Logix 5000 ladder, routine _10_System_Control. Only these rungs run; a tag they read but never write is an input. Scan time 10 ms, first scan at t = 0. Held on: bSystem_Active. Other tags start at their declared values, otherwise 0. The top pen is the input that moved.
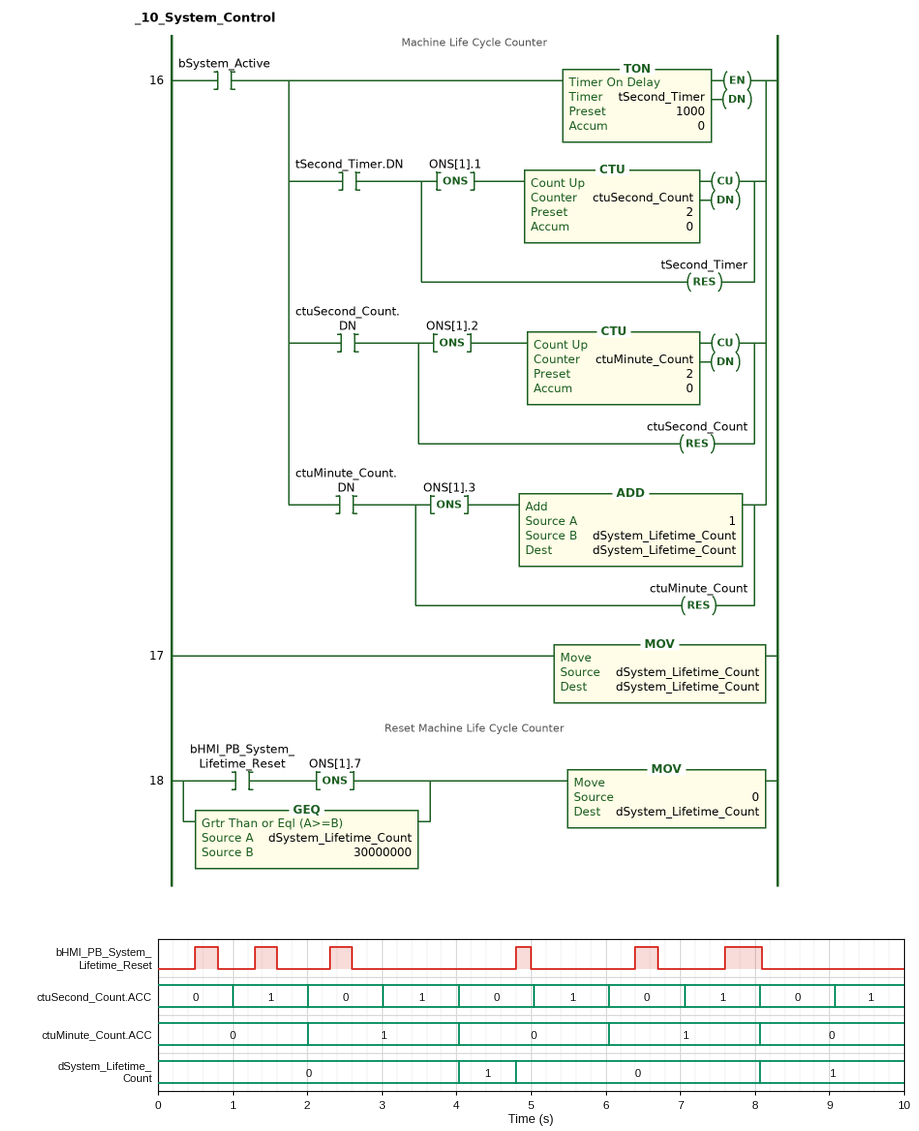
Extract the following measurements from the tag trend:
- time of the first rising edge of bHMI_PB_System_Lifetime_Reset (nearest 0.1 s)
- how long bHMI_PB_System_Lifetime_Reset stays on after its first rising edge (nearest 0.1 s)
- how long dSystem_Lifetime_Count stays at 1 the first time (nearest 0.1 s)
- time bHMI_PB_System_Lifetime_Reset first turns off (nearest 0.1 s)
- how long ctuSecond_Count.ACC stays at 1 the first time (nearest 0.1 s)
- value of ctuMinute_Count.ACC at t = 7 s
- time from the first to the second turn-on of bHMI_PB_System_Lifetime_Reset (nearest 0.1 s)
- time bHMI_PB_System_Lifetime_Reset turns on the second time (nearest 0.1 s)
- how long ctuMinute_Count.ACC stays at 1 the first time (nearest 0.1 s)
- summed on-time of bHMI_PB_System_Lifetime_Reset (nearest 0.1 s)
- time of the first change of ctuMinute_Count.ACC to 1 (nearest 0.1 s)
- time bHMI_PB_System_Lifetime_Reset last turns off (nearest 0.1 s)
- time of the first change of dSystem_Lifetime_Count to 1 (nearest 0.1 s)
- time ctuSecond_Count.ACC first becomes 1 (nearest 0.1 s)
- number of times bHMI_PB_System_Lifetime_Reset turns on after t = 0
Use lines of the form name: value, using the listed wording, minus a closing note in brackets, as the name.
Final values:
time of the first rising edge of bHMI_PB_System_Lifetime_Reset: 0.5 s
how long bHMI_PB_System_Lifetime_Reset stays on after its first rising edge: 0.3 s
how long dSystem_Lifetime_Count stays at 1 the first time: 0.8 s
time bHMI_PB_System_Lifetime_Reset first turns off: 0.8 s
how long ctuSecond_Count.ACC stays at 1 the first time: 1.0 s
value of ctuMinute_Count.ACC at t = 7 s: 1
time from the first to the second turn-on of bHMI_PB_System_Lifetime_Reset: 0.8 s
time bHMI_PB_System_Lifetime_Reset turns on the second time: 1.3 s
how long ctuMinute_Count.ACC stays at 1 the first time: 2.0 s
summed on-time of bHMI_PB_System_Lifetime_Reset: 1.9 s
time of the first change of ctuMinute_Count.ACC to 1: 2.0 s
time bHMI_PB_System_Lifetime_Reset last turns off: 8.1 s
time of the first change of dSystem_Lifetime_Count to 1: 4.0 s
time ctuSecond_Count.ACC first becomes 1: 1.0 s
number of times bHMI_PB_System_Lifetime_Reset turns on after t = 0: 6
